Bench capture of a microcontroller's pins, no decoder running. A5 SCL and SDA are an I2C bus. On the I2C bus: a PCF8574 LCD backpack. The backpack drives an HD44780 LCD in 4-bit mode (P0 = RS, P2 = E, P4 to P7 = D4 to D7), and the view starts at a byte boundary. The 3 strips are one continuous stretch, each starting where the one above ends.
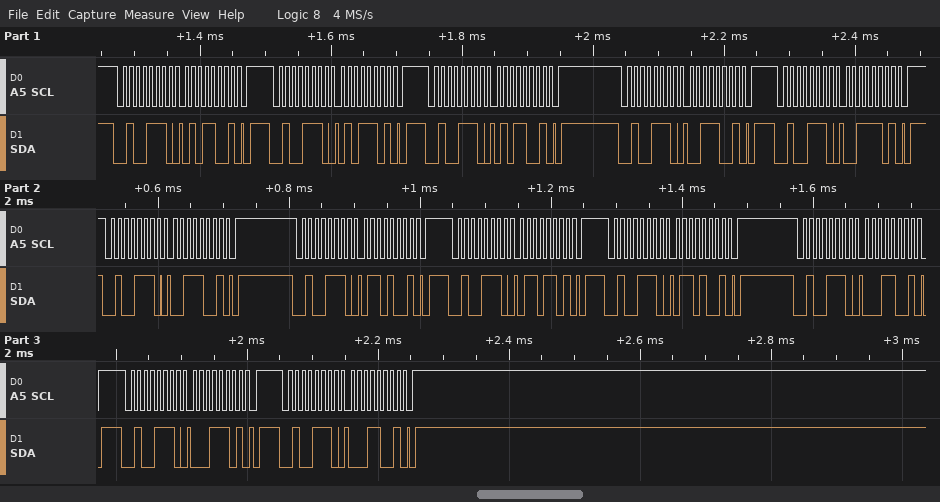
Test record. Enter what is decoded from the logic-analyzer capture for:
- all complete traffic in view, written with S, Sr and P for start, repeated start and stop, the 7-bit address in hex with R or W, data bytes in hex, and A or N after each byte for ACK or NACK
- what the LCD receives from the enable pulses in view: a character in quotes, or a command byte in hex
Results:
S 27W A 59 A P S 27W A 5D A P S 27W A 59 A P S 27W A 39 A P S 27W A 3D A P S 27W A 39 A P S 27W A 69 A P S 27W A 6D A P S 27W A 69 A P S 27W A 19 A P S 27W A 1D A P S 27W A 19 A P
'S' 'a'
